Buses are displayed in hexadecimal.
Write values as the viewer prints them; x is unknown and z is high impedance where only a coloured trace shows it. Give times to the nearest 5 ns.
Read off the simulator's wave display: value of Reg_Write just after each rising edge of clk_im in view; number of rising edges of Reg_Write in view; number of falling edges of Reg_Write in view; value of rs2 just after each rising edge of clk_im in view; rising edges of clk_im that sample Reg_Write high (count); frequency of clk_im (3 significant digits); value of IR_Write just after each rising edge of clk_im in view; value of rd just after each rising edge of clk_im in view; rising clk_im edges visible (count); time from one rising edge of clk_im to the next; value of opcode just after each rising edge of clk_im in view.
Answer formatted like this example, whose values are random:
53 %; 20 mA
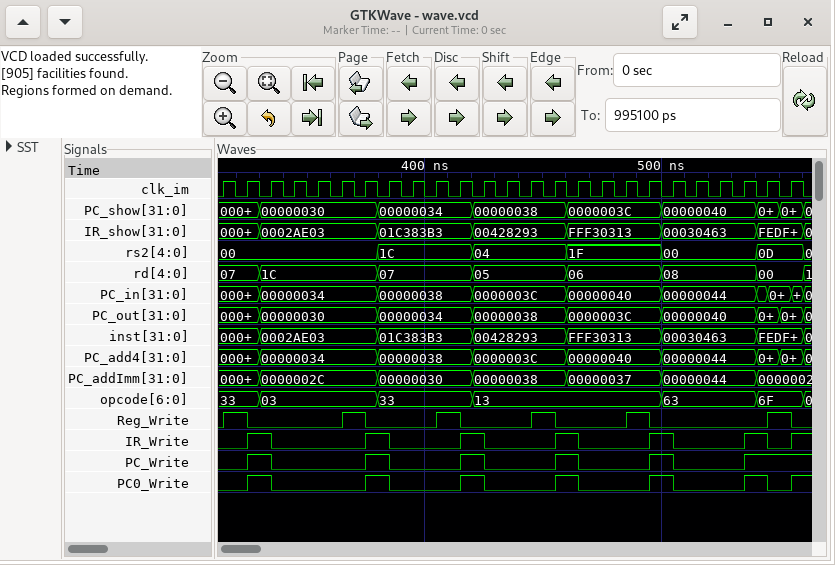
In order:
1 0 0 0 0 1 0 0 0 1 0 0 0 1 0 0 0 1 0 0 0 0 0 1 0; 6; 6; 00, 00, 00, 00, 00, 00, 00, 1C, 1C, 1C, 1C, 04, 04, 04, 04, 1F, 1F, 1F, 1F, 00, 00, 00, 00, 0D, 0D; 6; 100 MHz; 0 1 0 0 0 0 1 0 0 0 1 0 0 0 1 0 0 0 1 0 0 0 1 0 1; 07, 07, 1C, 1C, 1C, 1C, 1C, 07, 07, 07, 07, 05, 05, 05, 05, 06, 06, 06, 06, 08, 08, 08, 08, 00, 00; 25; 10 ns; 33, 33, 03, 03, 03, 03, 03, 33, 33, 33, 33, 13, 13, 13, 13, 13, 13, 13, 13, 63, 63, 63, 63, 6F, 6F
